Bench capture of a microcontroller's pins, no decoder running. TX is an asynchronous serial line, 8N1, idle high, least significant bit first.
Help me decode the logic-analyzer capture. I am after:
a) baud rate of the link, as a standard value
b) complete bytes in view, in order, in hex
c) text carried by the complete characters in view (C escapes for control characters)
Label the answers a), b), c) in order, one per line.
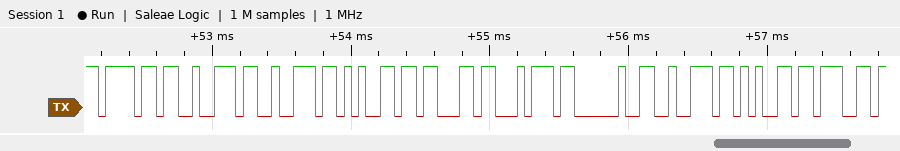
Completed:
a) 19200 baud
b) 6F 72 72 65 63 74 20 72 65 67
c) "orrect reg"
